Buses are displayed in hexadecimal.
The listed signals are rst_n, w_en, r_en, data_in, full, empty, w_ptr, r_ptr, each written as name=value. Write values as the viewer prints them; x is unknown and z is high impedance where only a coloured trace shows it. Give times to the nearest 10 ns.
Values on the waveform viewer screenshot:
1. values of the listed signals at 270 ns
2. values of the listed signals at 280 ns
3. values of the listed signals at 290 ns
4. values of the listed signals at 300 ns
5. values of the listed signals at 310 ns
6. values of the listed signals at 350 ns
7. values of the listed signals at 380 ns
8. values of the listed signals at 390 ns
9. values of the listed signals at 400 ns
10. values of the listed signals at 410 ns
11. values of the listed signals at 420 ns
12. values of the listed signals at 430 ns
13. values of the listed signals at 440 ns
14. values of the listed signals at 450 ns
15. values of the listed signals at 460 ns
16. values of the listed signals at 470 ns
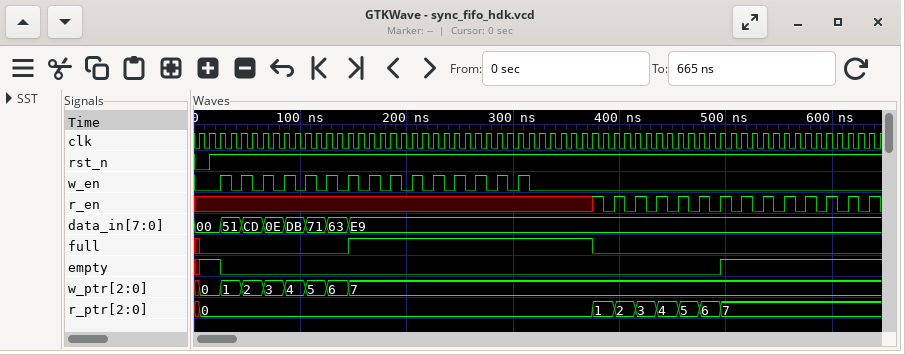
rst_n=1, w_en=1, r_en=x, data_in=E9, full=1, empty=0, w_ptr=7, r_ptr=0
rst_n=1, w_en=0, r_en=x, data_in=E9, full=1, empty=0, w_ptr=7, r_ptr=0
rst_n=1, w_en=1, r_en=x, data_in=E9, full=1, empty=0, w_ptr=7, r_ptr=0
rst_n=1, w_en=0, r_en=x, data_in=E9, full=1, empty=0, w_ptr=7, r_ptr=0
rst_n=1, w_en=1, r_en=x, data_in=E9, full=1, empty=0, w_ptr=7, r_ptr=0
rst_n=1, w_en=0, r_en=x, data_in=E9, full=1, empty=0, w_ptr=7, r_ptr=0
rst_n=1, w_en=0, r_en=1, data_in=E9, full=0, empty=0, w_ptr=7, r_ptr=1
rst_n=1, w_en=0, r_en=0, data_in=E9, full=0, empty=0, w_ptr=7, r_ptr=1
rst_n=1, w_en=0, r_en=1, data_in=E9, full=0, empty=0, w_ptr=7, r_ptr=2
rst_n=1, w_en=0, r_en=0, data_in=E9, full=0, empty=0, w_ptr=7, r_ptr=2
rst_n=1, w_en=0, r_en=1, data_in=E9, full=0, empty=0, w_ptr=7, r_ptr=3
rst_n=1, w_en=0, r_en=0, data_in=E9, full=0, empty=0, w_ptr=7, r_ptr=3
rst_n=1, w_en=0, r_en=1, data_in=E9, full=0, empty=0, w_ptr=7, r_ptr=4
rst_n=1, w_en=0, r_en=0, data_in=E9, full=0, empty=0, w_ptr=7, r_ptr=4
rst_n=1, w_en=0, r_en=1, data_in=E9, full=0, empty=0, w_ptr=7, r_ptr=5
rst_n=1, w_en=0, r_en=0, data_in=E9, full=0, empty=0, w_ptr=7, r_ptr=5
